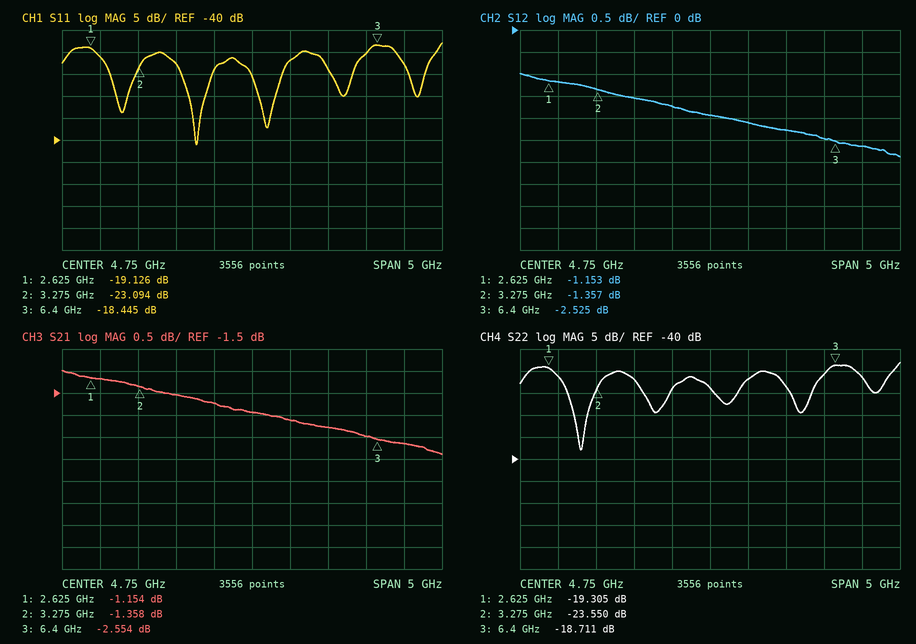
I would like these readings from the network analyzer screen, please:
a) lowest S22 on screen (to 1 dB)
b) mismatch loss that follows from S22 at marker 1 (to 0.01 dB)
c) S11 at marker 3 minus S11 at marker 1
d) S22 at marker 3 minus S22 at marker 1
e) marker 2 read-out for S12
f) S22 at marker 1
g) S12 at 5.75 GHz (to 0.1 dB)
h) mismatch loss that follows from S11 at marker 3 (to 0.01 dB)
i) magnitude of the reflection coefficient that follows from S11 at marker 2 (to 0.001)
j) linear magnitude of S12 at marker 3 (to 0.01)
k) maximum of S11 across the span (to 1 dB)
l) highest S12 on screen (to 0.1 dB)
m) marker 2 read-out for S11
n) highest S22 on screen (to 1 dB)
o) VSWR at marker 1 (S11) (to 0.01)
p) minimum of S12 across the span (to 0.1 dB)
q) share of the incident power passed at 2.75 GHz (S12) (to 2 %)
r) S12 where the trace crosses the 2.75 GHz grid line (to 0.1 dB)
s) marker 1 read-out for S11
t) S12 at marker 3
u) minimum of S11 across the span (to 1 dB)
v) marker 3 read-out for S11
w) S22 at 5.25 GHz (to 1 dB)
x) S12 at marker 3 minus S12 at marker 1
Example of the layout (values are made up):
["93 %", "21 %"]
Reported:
["-38 dB", "0.05 dB", "0.681 dB", "0.594 dB", "-1.357 dB", "-19.305 dB", "-2.3 dB", "0.06 dB", "0.070", "0.75", "-18 dB", "-1.0 dB", "-23.094 dB", "-18 dB", "1.25", "-2.9 dB", "76 %", "-1.2 dB", "-19.126 dB", "-2.525 dB", "-41 dB", "-18.445 dB", "-22 dB", "-1.372 dB"]
